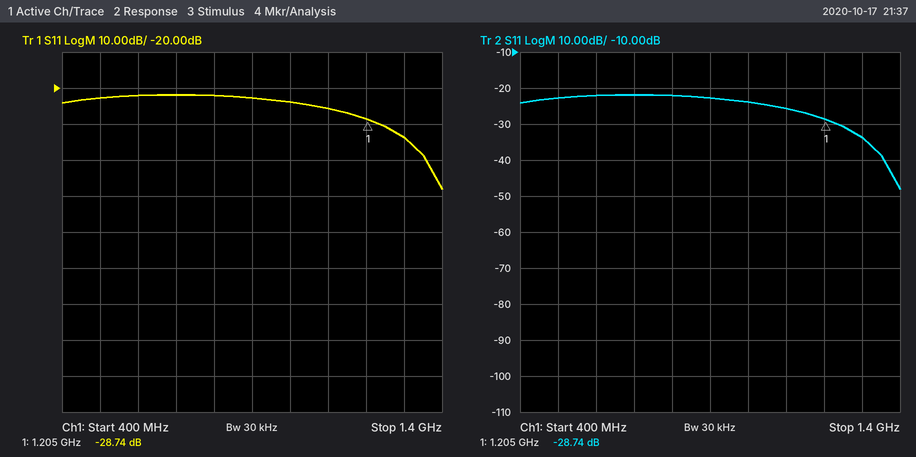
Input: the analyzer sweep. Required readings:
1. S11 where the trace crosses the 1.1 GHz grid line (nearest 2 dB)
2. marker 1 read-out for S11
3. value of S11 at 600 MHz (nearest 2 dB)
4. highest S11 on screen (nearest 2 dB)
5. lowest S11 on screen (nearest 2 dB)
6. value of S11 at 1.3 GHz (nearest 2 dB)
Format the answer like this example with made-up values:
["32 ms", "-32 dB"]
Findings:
["-26 dB", "-28.74 dB", "-22 dB", "-22 dB", "-48 dB", "-34 dB"]
